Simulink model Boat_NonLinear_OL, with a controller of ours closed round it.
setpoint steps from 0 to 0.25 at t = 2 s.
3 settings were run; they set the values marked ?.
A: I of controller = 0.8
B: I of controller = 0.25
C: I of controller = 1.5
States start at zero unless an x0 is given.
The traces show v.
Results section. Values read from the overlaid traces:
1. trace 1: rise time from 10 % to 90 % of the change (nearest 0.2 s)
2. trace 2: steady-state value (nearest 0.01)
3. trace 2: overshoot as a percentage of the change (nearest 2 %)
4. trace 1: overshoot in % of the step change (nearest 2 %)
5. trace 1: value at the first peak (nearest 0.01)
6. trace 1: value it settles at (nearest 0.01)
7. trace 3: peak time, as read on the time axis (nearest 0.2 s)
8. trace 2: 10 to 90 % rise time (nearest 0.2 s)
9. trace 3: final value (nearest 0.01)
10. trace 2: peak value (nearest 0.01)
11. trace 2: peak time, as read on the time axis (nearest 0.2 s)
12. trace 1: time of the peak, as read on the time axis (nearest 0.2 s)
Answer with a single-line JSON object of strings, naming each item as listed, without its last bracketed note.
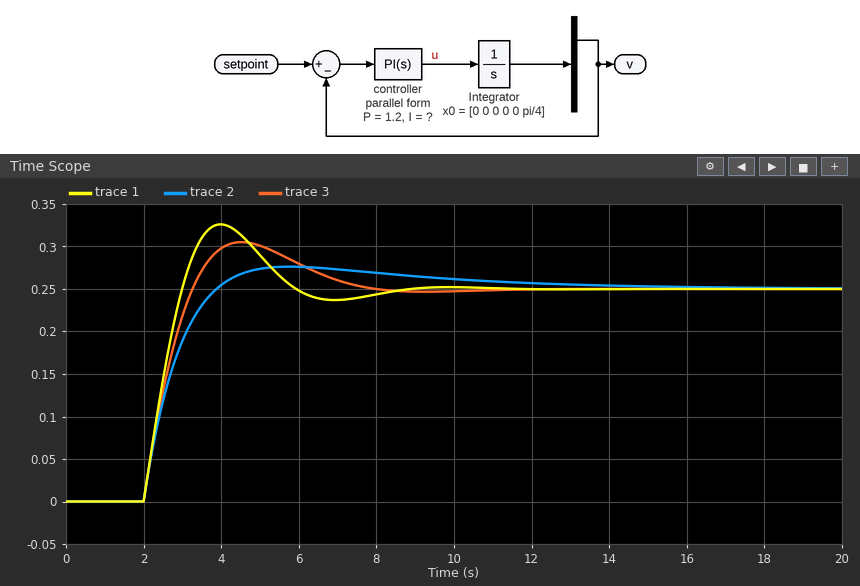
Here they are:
{"trace 1: rise time from 10 % to 90 % of the change": "0.8 s", "trace 2: steady-state value": "0.25", "trace 2: overshoot as a percentage of the change": "10 %", "trace 1: overshoot in % of the step change": "30 %", "trace 1: value at the first peak": "0.33", "trace 1: value it settles at": "0.25", "trace 3: peak time, as read on the time axis": "4.6 s", "trace 2: 10 to 90 % rise time": "1.4 s", "trace 3: final value": "0.25", "trace 2: peak value": "0.28", "trace 2: peak time, as read on the time axis": "5.8 s", "trace 1: time of the peak, as read on the time axis": "4.0 s"}
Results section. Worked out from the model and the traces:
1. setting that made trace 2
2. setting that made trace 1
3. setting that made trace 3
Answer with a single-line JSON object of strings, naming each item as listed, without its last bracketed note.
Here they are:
{"setting that made trace 2": "B", "setting that made trace 1": "C", "setting that made trace 3": "A"}
